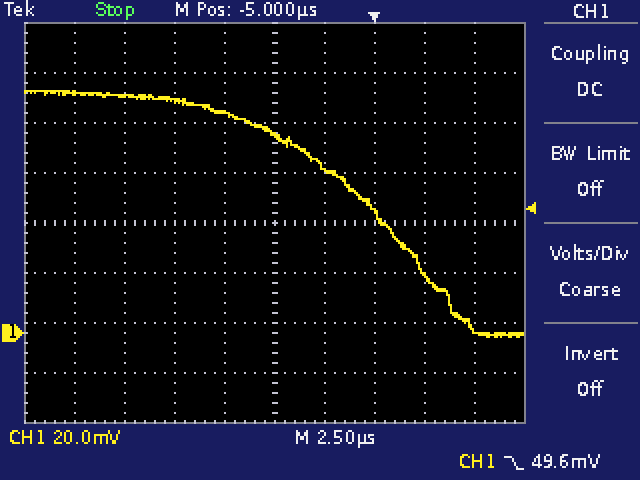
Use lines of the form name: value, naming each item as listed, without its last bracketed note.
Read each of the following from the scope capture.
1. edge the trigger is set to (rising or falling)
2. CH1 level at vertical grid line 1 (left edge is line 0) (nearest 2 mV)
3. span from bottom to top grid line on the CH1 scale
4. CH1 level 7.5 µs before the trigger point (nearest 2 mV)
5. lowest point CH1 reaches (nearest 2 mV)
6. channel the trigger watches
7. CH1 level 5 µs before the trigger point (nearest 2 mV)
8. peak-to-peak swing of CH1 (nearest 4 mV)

edge the trigger is set to: falling
CH1 level at vertical grid line 1 (left edge is line 0): 96 mV
span from bottom to top grid line on the CH1 scale: 160 mV
CH1 level 7.5 µs before the trigger point: 88 mV
lowest point CH1 reaches: -2 mV
channel the trigger watches: CH1
CH1 level 5 µs before the trigger point: 80 mV
peak-to-peak swing of CH1: 100 mV
